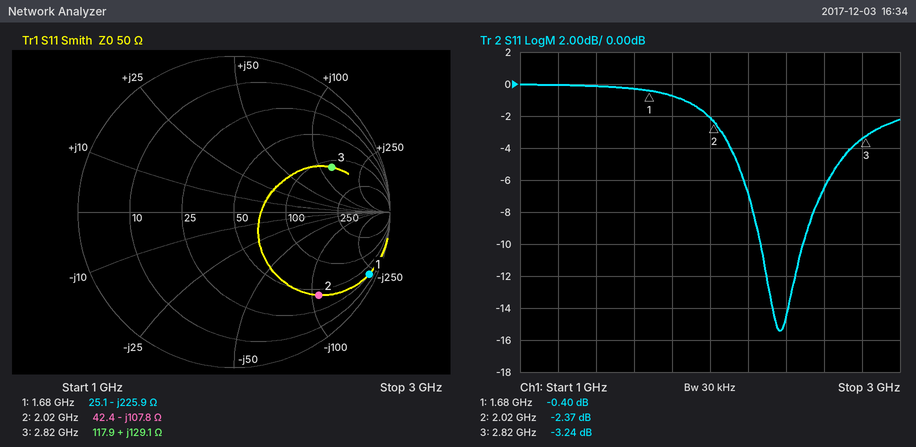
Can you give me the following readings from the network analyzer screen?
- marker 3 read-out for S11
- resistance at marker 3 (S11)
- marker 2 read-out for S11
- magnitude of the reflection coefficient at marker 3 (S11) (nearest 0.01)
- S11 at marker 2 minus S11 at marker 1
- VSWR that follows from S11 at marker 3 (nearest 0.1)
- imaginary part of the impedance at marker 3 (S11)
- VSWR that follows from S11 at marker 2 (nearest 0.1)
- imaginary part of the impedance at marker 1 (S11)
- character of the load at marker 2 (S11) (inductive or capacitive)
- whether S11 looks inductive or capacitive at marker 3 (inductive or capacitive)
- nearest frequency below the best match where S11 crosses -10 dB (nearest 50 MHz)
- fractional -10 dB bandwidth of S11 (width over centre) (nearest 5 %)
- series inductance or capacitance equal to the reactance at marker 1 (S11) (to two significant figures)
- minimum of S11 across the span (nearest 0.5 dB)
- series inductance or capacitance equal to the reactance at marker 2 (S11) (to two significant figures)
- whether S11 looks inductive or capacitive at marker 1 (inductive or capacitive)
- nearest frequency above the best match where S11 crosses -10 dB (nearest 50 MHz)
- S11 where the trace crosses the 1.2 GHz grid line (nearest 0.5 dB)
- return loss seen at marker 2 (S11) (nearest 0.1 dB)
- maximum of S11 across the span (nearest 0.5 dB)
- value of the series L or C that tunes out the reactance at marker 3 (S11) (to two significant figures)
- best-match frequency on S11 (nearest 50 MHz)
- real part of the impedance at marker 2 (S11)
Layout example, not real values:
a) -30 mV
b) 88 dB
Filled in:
a) -3.24 dB
b) 117.9 Ω
c) -2.37 dB
d) 0.69
e) -1.97 dB
f) 5.4
g) +129.1 Ω
h) 7.4
i) -225.9 Ω
j) capacitive
k) inductive
l) 2.25 GHz
m) 10 %
n) 420 fF
o) -15.5 dB
p) 730 fF
q) capacitive
r) 2.50 GHz
s) 0.0 dB
t) 2.4 dB
u) 0.0 dB
v) 440 fF
w) 2.35 GHz
x) 42.4 Ω
